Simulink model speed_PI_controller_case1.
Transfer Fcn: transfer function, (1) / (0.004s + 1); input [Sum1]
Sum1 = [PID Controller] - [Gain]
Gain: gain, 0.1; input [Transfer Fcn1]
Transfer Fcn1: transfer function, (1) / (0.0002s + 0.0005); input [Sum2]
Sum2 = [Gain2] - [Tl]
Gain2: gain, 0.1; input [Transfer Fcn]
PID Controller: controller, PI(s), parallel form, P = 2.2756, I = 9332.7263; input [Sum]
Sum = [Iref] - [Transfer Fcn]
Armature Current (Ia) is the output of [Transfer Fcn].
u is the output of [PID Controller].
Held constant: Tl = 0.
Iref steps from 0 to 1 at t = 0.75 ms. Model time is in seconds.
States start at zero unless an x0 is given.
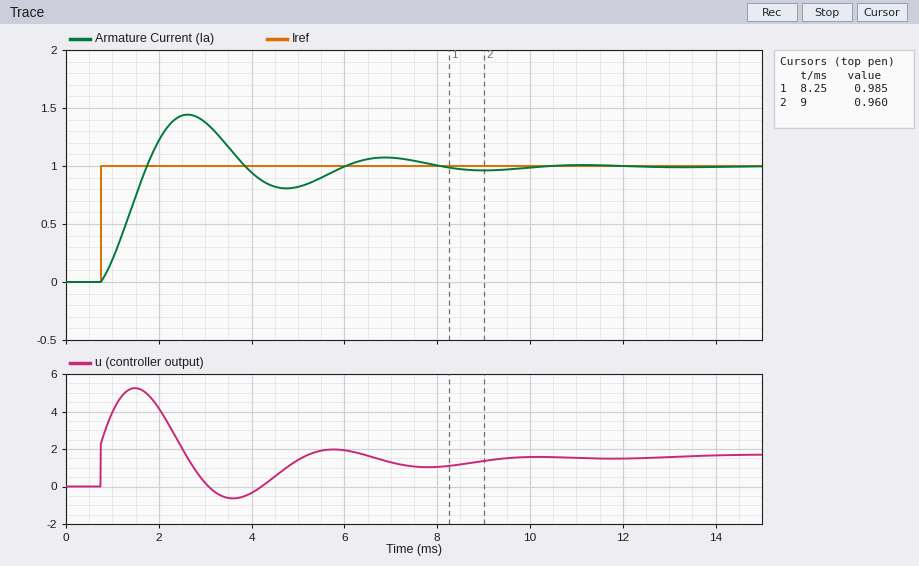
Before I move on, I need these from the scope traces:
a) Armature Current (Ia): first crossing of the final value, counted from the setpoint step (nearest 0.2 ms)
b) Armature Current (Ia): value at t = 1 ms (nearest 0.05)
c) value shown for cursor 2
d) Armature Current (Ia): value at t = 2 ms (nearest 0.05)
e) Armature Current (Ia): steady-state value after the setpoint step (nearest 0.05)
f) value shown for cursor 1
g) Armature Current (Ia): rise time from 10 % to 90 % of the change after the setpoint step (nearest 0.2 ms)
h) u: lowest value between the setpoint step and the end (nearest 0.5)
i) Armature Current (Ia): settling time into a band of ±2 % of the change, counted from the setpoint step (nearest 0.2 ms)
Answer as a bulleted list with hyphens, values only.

- 1.0 ms
- 0.20
- 0.960
- 1.20
- 1.00
- 0.985
- 0.8 ms
- -0.5
- 9.0 ms
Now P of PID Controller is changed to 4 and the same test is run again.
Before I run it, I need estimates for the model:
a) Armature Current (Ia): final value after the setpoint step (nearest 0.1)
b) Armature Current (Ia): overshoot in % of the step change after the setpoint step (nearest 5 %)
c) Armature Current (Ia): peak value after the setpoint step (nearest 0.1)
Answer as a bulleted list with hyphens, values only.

- 1.0
- 30 %
- 1.3
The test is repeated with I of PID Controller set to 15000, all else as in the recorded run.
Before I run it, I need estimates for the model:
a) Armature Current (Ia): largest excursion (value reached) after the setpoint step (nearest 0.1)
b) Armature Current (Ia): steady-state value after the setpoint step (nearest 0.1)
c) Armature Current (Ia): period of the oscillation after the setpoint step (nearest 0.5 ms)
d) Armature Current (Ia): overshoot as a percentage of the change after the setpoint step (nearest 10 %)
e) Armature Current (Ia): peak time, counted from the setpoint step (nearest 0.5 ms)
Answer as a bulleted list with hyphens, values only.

- 1.5
- 1.0
- 3.5 ms
- 50 %
- 1.5 ms
